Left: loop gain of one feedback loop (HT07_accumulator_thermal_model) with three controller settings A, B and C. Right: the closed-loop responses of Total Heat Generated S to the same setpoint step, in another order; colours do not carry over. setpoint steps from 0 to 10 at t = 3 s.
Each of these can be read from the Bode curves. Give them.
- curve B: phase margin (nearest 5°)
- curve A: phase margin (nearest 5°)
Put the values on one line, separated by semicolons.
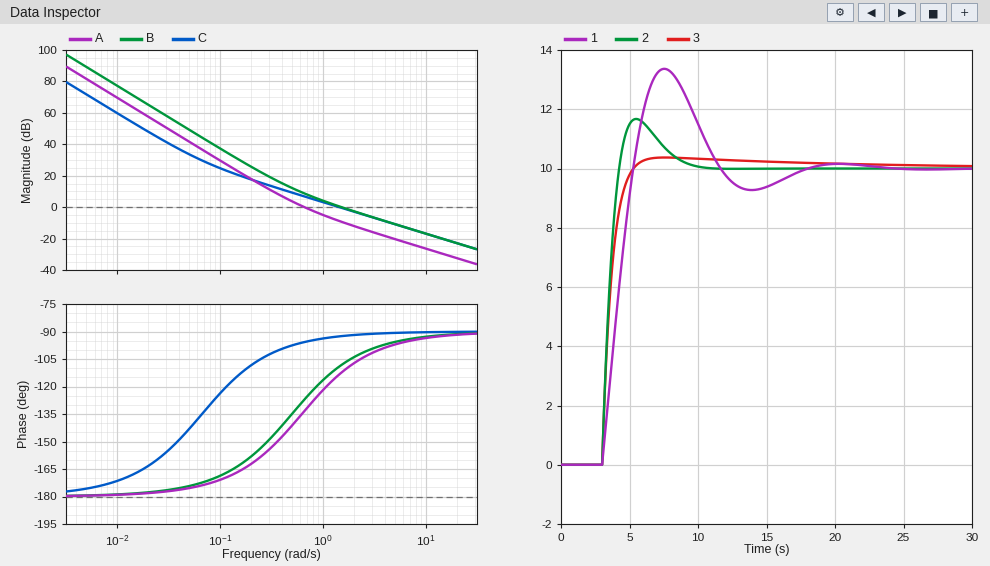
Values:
70°; 45°
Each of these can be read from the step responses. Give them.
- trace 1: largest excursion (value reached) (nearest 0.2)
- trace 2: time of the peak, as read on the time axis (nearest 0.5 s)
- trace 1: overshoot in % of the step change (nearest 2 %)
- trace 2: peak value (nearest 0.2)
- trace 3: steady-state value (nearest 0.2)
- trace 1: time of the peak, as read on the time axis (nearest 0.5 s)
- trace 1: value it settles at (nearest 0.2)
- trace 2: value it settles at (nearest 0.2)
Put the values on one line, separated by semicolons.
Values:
13.4; 5.5 s; 34 %; 11.6; 10.0; 7.5 s; 10.0; 10.0
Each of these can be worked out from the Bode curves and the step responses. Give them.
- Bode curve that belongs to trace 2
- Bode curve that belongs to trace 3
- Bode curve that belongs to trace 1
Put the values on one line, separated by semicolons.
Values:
B; C; A
